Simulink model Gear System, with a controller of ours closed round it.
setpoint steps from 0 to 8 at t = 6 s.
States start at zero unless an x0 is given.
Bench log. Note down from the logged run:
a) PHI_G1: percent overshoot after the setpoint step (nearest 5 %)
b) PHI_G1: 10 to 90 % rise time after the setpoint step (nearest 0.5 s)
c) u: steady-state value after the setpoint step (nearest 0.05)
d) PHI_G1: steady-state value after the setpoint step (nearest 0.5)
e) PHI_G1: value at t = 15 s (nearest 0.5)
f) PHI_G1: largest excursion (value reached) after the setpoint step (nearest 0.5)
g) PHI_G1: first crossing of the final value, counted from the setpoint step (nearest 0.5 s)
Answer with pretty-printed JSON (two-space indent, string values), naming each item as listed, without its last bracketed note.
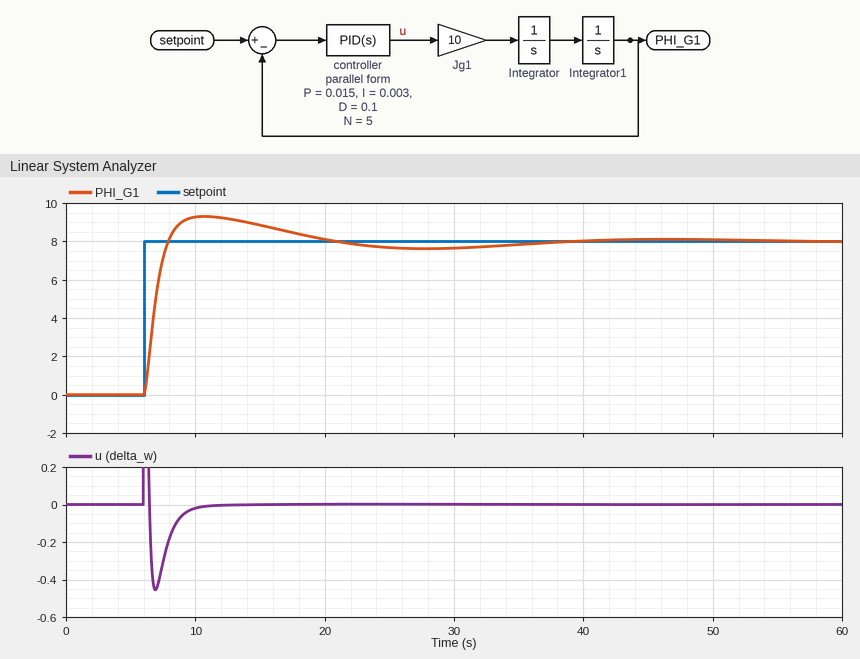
{
  "PHI_G1: percent overshoot after the setpoint step": "15 %",
  "PHI_G1: 10 to 90 % rise time after the setpoint step": "1.5 s",
  "u: steady-state value after the setpoint step": "0.00",
  "PHI_G1: steady-state value after the setpoint step": "8.0",
  "PHI_G1: value at t = 15 s": "9.0",
  "PHI_G1: largest excursion (value reached) after the setpoint step": "9.5",
  "PHI_G1: first crossing of the final value, counted from the setpoint step": "2.0 s"
}
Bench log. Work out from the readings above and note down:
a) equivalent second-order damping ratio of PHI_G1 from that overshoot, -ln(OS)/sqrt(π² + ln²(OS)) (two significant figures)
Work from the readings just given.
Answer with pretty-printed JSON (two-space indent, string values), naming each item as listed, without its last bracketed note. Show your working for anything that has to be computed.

{
  "equivalent second-order damping ratio of PHI_G1 from that overshoot, -ln(OS)/sqrt(π² + ln²(OS))": "ln(0.15) = -1.897; 1.897 / sqrt(9.870 + 3.599) = 0.52"
}
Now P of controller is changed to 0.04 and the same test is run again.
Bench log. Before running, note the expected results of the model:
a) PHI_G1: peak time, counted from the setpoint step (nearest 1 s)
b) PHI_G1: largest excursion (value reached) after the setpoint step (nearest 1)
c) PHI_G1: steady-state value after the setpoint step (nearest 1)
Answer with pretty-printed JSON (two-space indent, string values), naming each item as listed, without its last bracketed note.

{
  "PHI_G1: peak time, counted from the setpoint step": "3 s",
  "PHI_G1: largest excursion (value reached) after the setpoint step": "10",
  "PHI_G1: steady-state value after the setpoint step": "8"
}
